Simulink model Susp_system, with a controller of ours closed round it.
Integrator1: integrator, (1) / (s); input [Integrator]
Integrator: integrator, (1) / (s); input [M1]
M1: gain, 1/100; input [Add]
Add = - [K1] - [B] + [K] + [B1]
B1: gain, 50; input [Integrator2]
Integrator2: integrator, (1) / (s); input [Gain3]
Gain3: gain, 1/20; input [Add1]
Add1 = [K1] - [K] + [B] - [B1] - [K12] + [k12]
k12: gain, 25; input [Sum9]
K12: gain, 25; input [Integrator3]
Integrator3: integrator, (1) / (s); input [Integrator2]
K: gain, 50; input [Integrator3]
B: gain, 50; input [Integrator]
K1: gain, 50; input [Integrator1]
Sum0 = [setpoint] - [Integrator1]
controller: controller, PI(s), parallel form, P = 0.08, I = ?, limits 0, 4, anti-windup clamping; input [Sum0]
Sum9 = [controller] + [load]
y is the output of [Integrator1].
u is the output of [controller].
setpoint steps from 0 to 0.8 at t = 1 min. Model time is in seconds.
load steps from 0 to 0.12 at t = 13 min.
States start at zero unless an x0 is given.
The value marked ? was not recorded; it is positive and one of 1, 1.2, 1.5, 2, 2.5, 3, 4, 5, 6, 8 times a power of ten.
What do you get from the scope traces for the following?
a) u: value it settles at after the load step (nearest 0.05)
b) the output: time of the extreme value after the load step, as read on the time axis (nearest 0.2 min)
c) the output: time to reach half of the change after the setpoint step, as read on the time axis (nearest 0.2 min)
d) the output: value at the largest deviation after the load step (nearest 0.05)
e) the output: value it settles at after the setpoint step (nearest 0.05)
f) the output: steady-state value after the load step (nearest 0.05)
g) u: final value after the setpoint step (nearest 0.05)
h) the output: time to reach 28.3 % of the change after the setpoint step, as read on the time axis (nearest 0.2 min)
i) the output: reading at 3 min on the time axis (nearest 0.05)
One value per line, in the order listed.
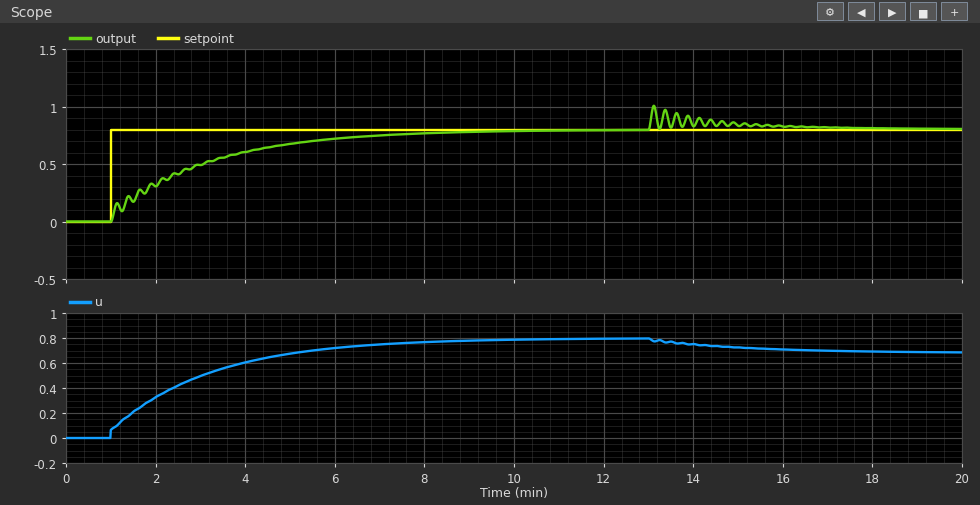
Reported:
0.70
13.2 min
2.4 min
1.00
0.80
0.80
0.80
1.6 min
0.50
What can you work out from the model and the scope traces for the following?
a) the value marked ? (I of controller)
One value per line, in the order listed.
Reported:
0.008
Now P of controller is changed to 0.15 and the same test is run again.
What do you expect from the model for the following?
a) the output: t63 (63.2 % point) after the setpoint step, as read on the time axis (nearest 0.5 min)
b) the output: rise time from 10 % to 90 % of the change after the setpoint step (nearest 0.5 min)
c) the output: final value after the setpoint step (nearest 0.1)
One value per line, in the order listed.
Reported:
3.0 min
5.0 min
0.8
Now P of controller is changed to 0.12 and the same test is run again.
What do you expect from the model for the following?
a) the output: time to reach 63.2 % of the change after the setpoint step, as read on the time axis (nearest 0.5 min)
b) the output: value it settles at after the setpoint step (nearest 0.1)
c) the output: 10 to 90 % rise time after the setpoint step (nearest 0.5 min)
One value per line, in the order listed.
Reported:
3.0 min
0.8
5.0 min
